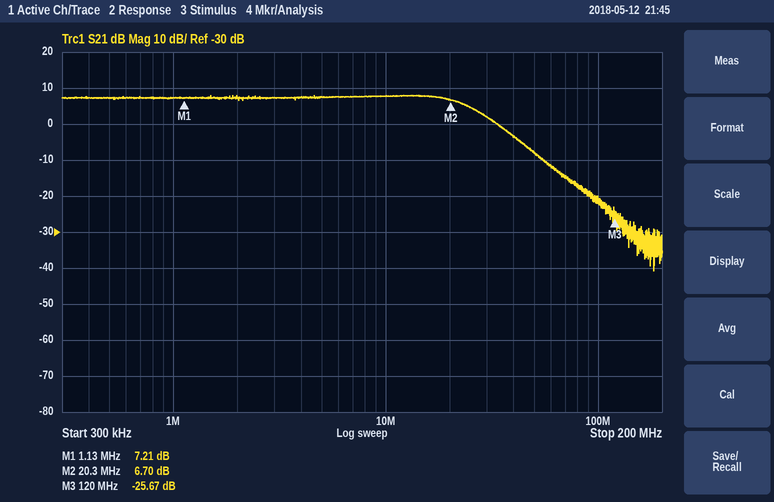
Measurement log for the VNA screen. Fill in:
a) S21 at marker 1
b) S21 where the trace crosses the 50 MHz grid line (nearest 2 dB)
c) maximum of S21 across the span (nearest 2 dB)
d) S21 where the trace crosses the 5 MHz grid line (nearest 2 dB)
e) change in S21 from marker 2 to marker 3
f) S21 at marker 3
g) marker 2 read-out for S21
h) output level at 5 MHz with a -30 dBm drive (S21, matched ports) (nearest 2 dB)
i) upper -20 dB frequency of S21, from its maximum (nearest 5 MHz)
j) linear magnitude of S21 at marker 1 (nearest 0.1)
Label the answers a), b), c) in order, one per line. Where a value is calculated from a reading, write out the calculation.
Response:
a) 7.21 dB
b) -8 dB
c) 8 dB
d) 8 dB
e) -25.67 − (6.7) = -32.37 dB
f) -25.67 dB
g) 6.70 dB
h) -30 dBm + (8 dB) = -22 dBm
i) 60 MHz
j) 10^(7.21/20) ≈ 2.3
